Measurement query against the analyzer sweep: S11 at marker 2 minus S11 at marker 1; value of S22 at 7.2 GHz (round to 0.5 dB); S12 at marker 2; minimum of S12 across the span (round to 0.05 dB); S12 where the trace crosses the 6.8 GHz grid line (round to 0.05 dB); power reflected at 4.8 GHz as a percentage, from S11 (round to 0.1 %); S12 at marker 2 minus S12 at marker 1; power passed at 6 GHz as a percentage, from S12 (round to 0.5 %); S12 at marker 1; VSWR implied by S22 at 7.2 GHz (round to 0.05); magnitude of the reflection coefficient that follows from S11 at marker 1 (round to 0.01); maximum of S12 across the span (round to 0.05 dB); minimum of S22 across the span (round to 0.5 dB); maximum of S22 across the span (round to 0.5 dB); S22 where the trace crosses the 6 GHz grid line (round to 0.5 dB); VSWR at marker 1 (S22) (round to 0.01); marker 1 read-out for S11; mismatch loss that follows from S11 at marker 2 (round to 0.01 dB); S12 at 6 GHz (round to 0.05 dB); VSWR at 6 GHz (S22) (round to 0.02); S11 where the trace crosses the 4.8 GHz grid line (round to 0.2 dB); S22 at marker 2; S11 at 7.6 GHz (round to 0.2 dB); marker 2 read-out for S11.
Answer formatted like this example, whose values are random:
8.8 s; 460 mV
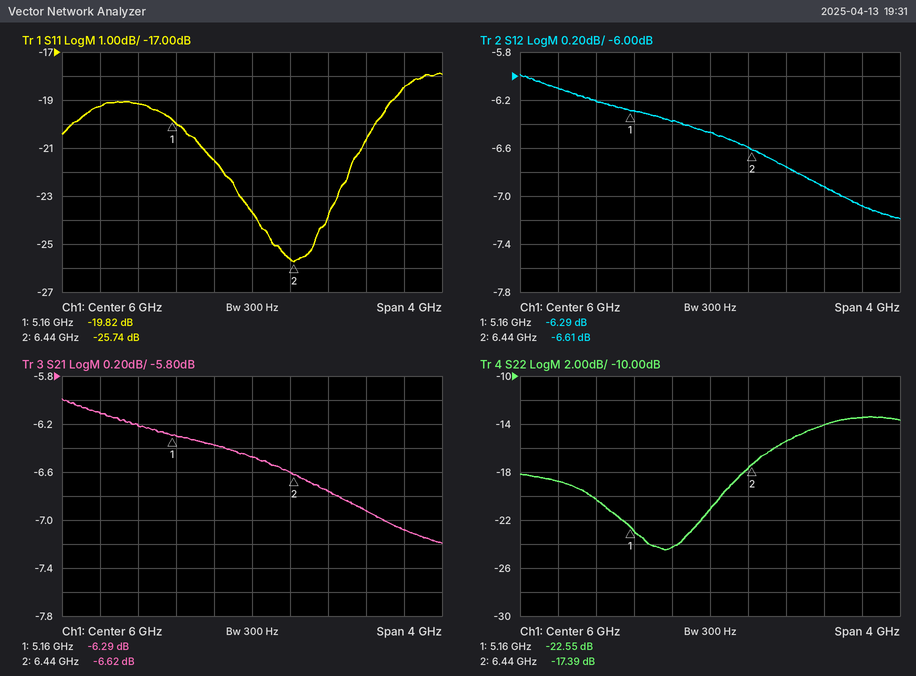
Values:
-5.92 dB; -14.0 dB; -6.61 dB; -7.20 dB; -6.75 dB; 1.2 %; -0.32 dB; 22.5 %; -6.29 dB; 1.50; 0.10; -6.00 dB; -24.5 dB; -13.5 dB; -21.0 dB; 1.16; -19.82 dB; 0.01 dB; -6.45 dB; 1.20; -19.2 dB; -17.39 dB; -18.4 dB; -25.74 dB
